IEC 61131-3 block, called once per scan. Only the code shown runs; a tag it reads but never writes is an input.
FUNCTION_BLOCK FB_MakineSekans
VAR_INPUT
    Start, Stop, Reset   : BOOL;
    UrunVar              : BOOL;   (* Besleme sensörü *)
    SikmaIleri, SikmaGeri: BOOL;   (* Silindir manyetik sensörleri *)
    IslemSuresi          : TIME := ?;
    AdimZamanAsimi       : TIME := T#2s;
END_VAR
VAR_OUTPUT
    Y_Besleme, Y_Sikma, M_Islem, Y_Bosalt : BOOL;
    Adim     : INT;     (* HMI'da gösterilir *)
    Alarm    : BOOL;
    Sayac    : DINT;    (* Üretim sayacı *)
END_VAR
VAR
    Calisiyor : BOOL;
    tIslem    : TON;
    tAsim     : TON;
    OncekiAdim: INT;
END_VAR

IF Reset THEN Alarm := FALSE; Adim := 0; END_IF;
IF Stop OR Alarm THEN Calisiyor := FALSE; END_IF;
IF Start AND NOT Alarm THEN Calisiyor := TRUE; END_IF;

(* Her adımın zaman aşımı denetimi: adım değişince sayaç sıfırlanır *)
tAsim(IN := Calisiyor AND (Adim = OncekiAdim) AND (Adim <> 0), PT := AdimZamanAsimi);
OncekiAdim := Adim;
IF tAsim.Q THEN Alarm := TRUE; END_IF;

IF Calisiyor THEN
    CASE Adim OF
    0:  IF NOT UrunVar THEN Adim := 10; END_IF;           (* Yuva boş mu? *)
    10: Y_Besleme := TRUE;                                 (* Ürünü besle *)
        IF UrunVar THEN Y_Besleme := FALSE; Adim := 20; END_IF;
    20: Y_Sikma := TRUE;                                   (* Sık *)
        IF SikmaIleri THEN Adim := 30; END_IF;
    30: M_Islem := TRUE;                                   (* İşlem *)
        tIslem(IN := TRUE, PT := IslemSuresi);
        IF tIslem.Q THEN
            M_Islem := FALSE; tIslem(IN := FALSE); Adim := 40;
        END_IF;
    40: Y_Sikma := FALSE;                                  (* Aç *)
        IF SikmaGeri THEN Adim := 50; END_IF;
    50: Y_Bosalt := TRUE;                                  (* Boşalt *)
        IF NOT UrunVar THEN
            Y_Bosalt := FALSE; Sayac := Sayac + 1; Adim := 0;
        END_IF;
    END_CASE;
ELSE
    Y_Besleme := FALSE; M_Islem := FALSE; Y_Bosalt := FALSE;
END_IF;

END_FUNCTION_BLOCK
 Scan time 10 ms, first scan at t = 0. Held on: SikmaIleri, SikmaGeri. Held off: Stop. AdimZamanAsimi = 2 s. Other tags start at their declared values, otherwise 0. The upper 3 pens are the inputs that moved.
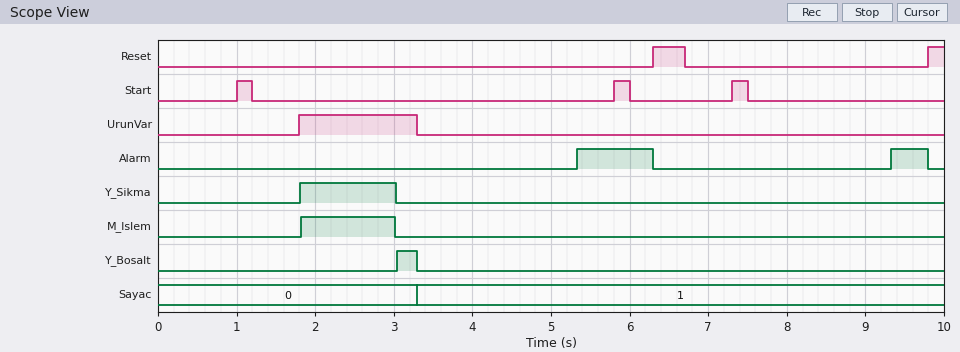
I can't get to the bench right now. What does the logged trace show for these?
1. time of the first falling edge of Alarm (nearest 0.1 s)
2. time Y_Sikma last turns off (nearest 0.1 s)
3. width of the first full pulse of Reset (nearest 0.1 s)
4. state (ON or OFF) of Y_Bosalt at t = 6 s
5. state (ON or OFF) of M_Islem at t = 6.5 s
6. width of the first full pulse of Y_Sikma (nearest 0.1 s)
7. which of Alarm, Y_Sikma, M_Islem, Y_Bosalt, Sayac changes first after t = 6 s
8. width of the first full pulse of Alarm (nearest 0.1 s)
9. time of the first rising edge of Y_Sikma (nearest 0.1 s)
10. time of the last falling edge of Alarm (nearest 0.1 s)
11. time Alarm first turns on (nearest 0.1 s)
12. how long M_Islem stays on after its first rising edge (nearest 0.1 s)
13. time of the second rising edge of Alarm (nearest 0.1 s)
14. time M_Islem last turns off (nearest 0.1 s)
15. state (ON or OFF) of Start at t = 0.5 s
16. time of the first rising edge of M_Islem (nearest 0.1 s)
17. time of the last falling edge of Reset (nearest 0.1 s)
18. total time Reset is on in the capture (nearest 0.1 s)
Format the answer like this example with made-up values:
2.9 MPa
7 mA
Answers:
6.3 s
3.0 s
0.4 s
OFF
OFF
1.2 s
Alarm
1.0 s
1.8 s
9.8 s
5.3 s
1.2 s
9.3 s
3.0 s
OFF
1.8 s
6.7 s
0.6 s
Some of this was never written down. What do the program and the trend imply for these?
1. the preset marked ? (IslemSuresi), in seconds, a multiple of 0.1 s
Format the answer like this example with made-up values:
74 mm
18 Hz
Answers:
1.2 s
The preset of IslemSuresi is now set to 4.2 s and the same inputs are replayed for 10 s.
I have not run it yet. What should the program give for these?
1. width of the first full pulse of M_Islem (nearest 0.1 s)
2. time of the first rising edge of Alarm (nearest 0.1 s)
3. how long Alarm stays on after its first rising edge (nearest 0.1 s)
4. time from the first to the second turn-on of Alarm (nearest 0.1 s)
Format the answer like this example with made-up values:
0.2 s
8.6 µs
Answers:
2.0 s
3.8 s
2.5 s
5.5 s
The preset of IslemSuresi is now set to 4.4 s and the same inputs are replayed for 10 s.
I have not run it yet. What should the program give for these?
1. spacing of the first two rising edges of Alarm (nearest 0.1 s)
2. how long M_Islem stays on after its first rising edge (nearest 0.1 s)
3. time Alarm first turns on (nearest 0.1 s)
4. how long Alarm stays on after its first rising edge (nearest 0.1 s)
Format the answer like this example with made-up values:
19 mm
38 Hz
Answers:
5.5 s
2.0 s
3.8 s
2.5 s
